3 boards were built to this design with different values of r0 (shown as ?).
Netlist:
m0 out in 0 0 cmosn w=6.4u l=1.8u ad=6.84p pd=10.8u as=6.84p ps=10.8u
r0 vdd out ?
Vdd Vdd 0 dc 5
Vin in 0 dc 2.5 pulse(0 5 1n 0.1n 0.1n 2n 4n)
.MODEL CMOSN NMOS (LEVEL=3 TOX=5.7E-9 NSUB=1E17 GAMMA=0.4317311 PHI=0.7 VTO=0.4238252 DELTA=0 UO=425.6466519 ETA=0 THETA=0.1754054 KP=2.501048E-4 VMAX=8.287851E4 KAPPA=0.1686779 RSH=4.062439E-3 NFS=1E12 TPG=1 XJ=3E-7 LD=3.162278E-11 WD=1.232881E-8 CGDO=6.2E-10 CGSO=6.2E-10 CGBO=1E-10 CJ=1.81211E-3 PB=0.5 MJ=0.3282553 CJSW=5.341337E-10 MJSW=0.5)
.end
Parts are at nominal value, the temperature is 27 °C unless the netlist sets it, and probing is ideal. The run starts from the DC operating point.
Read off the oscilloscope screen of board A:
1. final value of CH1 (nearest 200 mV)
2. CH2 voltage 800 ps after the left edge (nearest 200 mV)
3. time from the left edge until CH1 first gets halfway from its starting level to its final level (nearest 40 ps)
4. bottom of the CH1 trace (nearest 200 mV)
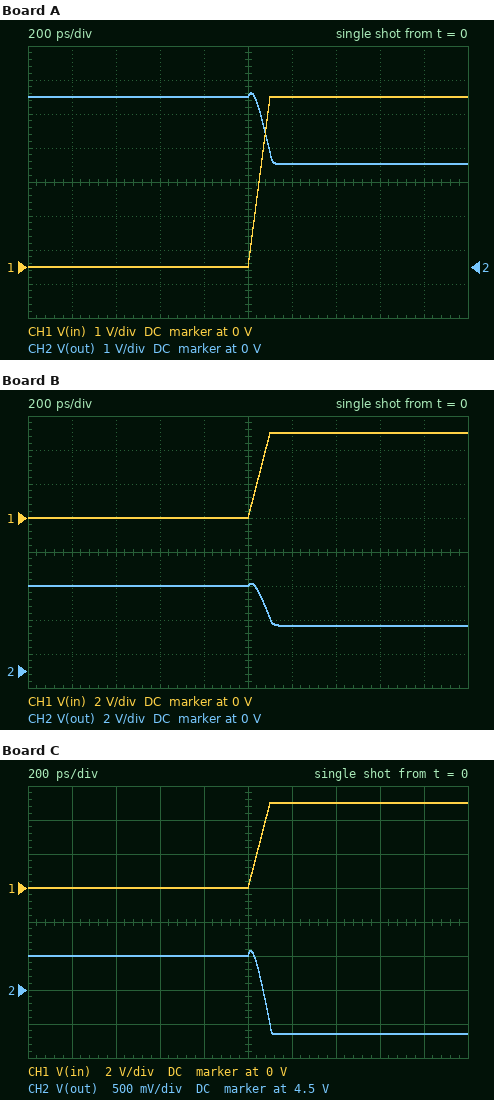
5.0 V
5.0 V
1.04 ns
0 V
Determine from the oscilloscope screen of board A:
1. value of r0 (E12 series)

680 Ω
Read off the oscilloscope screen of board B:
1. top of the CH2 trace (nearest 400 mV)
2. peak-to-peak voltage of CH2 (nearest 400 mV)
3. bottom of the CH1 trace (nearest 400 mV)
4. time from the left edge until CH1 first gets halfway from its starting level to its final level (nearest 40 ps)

5.2 V
2.4 V
0 V
1.04 ns
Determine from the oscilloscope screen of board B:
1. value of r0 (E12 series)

820 Ω
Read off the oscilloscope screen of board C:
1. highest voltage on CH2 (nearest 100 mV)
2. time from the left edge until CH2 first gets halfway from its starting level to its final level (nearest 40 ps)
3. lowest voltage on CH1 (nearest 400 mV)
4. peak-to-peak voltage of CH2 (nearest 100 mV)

5.1 V
1.08 ns
0 V
1.2 V
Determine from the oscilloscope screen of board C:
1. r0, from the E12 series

390 Ω
